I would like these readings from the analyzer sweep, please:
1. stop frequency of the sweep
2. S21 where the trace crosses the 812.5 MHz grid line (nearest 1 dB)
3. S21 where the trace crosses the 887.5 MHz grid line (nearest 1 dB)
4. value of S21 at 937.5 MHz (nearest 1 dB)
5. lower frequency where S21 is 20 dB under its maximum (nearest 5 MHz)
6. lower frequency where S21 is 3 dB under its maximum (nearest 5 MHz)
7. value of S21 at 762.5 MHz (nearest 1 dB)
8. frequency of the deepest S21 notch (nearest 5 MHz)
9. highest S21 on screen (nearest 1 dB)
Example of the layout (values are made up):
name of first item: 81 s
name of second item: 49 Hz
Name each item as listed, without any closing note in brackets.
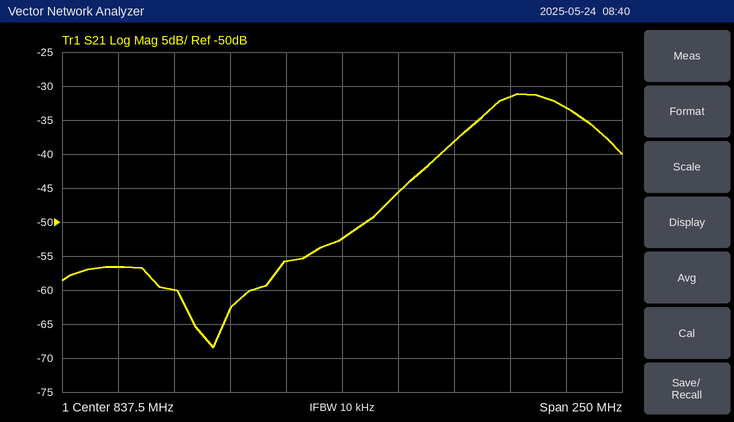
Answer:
stop frequency of the sweep: 962.5 MHz
S21 where the trace crosses the 812.5 MHz grid line: -56 dB
S21 where the trace crosses the 887.5 MHz grid line: -38 dB
value of S21 at 937.5 MHz: -33 dB
lower frequency where S21 is 20 dB under its maximum: 845 MHz
lower frequency where S21 is 3 dB under its maximum: 900 MHz
value of S21 at 762.5 MHz: -60 dB
frequency of the deepest S21 notch: 780 MHz
highest S21 on screen: -31 dB
